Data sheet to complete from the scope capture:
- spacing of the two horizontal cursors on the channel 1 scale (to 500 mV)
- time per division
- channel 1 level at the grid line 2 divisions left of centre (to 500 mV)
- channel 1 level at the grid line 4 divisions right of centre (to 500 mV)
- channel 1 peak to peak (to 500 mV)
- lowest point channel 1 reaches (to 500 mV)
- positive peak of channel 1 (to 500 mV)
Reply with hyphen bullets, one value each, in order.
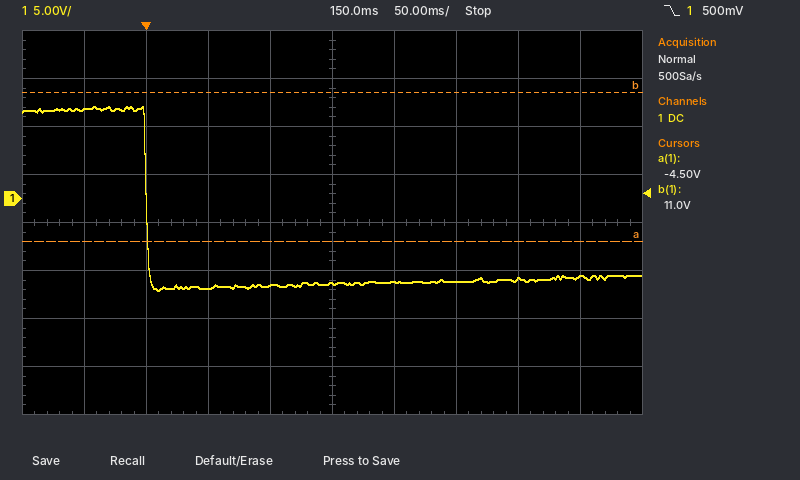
- 15.5 V
- 50 ms
- -9.5 V
- -8.0 V
- 19.0 V
- -9.5 V
- 9.5 V
